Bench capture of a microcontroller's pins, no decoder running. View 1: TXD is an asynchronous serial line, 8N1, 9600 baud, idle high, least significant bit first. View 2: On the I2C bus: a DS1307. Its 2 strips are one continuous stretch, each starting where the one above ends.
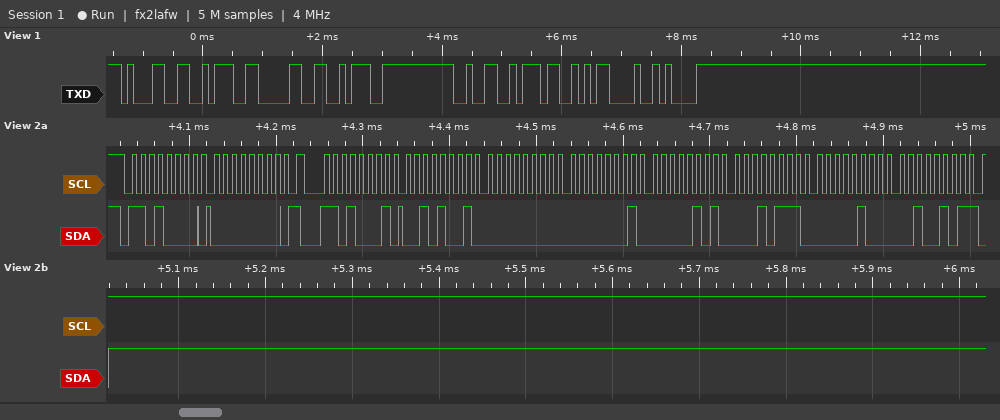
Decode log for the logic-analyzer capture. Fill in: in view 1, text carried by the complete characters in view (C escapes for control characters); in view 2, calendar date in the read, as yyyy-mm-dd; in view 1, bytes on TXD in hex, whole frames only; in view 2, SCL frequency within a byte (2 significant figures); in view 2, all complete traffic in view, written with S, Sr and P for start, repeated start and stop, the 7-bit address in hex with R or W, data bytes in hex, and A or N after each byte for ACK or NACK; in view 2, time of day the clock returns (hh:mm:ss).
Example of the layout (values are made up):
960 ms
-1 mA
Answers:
"1:0:27\r\n"
2025-04-17
31 3A 30 3A 32 37 0D 0A
100 kHz
S 68W A 00 A Sr 68R A 29 A 00 A 01 A 05 A 17 A 04 A 25 N P
01:00:29
